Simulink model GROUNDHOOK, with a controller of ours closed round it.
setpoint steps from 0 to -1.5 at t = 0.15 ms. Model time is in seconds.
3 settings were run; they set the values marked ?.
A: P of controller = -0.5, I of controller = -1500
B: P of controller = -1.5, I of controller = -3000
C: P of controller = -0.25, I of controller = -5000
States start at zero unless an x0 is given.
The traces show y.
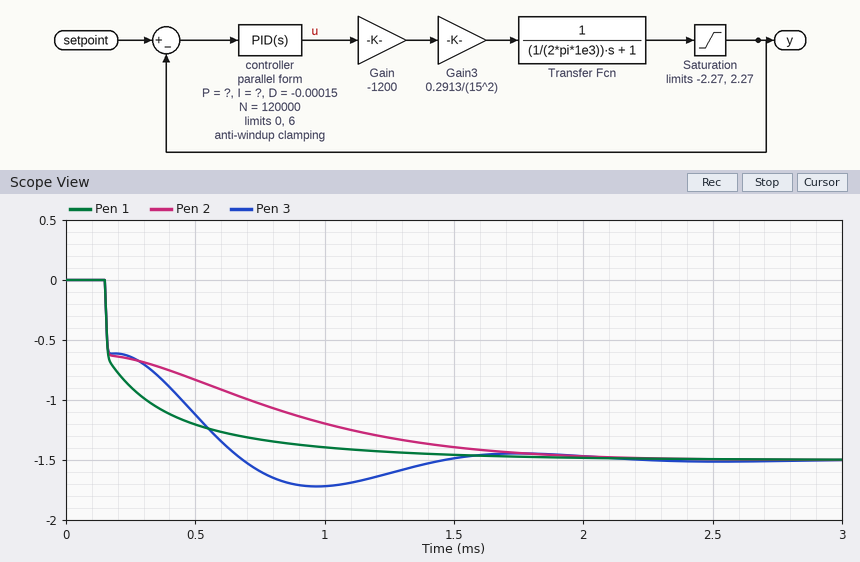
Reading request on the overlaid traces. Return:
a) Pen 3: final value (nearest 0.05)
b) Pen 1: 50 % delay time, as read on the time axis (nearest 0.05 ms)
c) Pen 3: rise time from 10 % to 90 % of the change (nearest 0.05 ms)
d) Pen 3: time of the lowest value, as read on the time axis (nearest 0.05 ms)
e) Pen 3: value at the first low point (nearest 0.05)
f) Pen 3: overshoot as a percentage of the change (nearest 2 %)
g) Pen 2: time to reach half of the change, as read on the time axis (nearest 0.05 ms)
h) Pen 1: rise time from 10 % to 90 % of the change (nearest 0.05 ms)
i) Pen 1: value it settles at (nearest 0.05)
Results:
-1.50
0.20 ms
0.45 ms
0.95 ms
-1.70
14 %
0.40 ms
0.65 ms
-1.50
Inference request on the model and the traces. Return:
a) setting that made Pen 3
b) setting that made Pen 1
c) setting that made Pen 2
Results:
C
B
A
